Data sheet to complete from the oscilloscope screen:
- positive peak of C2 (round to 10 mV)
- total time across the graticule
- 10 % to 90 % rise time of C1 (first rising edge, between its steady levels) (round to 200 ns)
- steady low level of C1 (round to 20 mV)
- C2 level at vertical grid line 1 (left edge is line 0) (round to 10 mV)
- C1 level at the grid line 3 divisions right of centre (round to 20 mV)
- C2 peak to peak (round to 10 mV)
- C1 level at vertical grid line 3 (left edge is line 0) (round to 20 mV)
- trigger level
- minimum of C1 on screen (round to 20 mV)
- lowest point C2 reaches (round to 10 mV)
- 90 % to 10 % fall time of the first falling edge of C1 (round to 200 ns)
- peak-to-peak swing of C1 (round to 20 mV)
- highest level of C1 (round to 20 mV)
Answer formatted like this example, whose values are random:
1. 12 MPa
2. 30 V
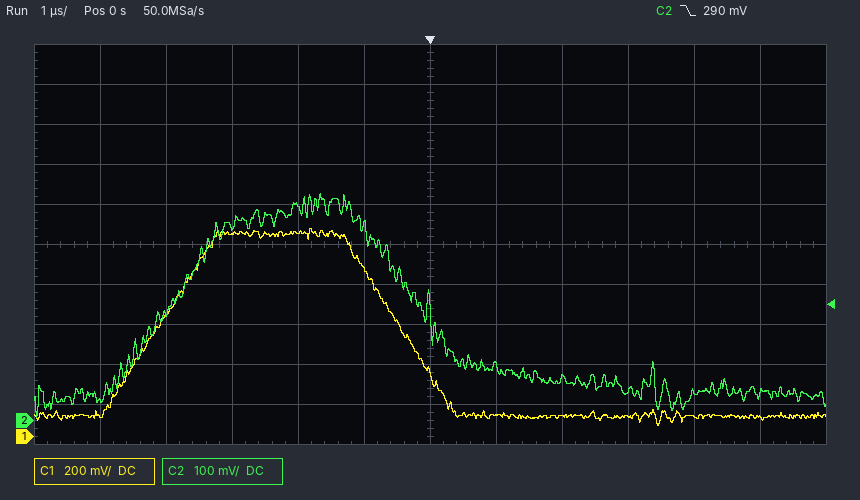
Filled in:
1. 570 mV
2. 12 µs
3. 1.4 µs
4. 100 mV
5. 50 mV
6. 100 mV
7. 560 mV
8. 1.02 V
9. 290 mV
10. 60 mV
11. 10 mV
12. 1.4 µs
13. 980 mV
14. 1.04 V
